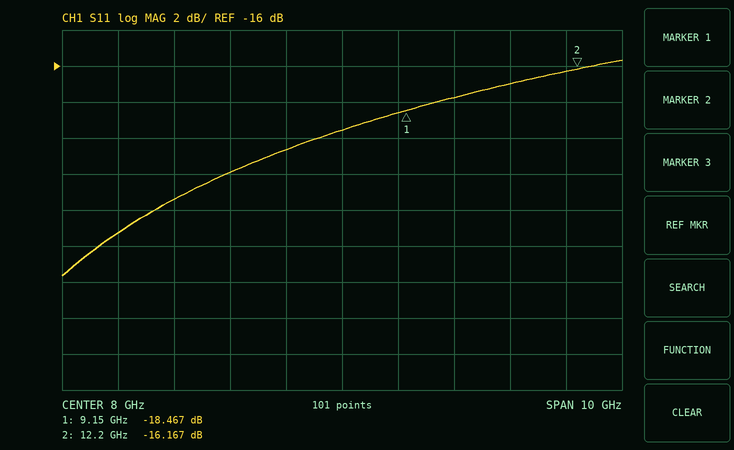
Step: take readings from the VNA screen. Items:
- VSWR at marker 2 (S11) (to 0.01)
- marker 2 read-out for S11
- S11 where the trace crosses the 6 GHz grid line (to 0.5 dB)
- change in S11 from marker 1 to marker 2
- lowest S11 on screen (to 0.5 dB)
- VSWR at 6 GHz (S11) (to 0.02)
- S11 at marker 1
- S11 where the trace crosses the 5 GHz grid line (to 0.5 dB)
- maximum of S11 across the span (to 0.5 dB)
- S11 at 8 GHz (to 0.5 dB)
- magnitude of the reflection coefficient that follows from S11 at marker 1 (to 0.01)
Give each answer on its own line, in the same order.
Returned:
1.37
-16.167 dB
-22.0 dB
2.300 dB
-27.5 dB
1.18
-18.467 dB
-23.5 dB
-15.5 dB
-19.5 dB
0.12
